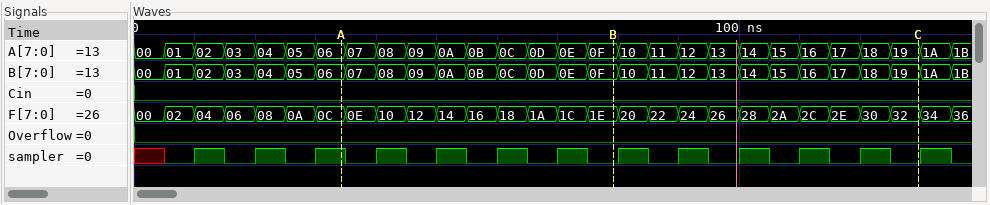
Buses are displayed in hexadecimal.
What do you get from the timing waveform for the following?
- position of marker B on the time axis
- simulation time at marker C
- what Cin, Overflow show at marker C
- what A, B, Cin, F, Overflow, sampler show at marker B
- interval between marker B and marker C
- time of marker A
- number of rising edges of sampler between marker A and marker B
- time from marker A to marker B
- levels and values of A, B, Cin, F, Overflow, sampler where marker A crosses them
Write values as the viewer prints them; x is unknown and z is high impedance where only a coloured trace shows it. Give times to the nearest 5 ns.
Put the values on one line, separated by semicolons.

80 ns; 130 ns; Cin=0, Overflow=0; A=0F, B=0F, Cin=0, F=1E, Overflow=0, sampler=0; 50 ns; 35 ns; 4; 45 ns; A=06, B=06, Cin=0, F=0C, Overflow=0, sampler=1
